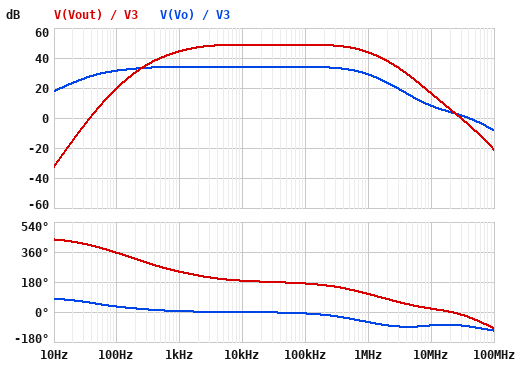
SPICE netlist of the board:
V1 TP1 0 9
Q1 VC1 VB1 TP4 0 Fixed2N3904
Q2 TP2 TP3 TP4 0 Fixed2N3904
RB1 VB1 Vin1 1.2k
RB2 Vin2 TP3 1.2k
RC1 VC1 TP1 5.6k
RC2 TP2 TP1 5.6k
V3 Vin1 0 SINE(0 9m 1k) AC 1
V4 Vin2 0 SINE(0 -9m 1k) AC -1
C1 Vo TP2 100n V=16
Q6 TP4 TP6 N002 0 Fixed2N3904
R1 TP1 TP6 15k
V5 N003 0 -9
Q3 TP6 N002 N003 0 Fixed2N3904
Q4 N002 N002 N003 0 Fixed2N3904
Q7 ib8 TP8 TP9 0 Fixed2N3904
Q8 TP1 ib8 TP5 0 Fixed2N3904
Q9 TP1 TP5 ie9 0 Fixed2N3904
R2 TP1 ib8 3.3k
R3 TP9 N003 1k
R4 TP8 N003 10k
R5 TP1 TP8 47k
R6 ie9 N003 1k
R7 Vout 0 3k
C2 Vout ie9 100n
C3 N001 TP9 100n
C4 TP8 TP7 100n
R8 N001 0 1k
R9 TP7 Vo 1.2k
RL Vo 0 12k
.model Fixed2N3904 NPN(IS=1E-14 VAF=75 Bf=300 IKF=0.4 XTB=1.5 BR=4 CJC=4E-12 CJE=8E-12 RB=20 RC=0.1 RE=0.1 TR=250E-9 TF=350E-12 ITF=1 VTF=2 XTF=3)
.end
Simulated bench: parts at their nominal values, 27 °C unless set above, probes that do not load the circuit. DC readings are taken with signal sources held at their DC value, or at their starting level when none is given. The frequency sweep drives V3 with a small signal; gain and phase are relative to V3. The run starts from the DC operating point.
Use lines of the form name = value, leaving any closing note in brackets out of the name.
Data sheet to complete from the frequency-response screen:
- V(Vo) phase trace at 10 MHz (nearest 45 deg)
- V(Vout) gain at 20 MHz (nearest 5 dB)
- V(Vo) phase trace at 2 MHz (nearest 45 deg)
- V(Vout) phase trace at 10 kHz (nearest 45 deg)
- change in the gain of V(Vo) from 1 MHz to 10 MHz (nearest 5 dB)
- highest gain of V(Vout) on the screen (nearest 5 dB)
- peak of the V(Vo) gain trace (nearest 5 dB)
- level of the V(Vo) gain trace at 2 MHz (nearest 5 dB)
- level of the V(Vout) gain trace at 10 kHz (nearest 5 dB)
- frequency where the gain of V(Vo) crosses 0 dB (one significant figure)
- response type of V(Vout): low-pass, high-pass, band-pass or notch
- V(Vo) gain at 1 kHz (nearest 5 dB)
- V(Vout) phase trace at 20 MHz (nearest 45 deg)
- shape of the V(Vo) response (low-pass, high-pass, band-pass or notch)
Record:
V(Vo) phase trace at 10 MHz = -90 deg
V(Vout) gain at 20 MHz = 5 dB
V(Vo) phase trace at 2 MHz = -90 deg
V(Vout) phase trace at 10 kHz = 180 deg
change in the gain of V(Vo) from 1 MHz to 10 MHz = -20 dB
highest gain of V(Vout) on the screen = 50 dB
peak of the V(Vo) gain trace = 35 dB
level of the V(Vo) gain trace at 2 MHz = 25 dB
level of the V(Vout) gain trace at 10 kHz = 50 dB
frequency where the gain of V(Vo) crosses 0 dB = 40 MHz
response type of V(Vout): low-pass, high-pass, band-pass or notch = band-pass
V(Vo) gain at 1 kHz = 35 dB
V(Vout) phase trace at 20 MHz = 0 deg
shape of the V(Vo) response = band-pass
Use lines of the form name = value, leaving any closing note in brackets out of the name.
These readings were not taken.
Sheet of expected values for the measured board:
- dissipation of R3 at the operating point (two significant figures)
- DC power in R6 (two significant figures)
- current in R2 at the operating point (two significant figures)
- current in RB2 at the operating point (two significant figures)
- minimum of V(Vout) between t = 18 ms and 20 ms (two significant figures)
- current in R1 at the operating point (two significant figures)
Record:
dissipation of R3 at the operating point = 5.9 mW
DC power in R6 = 77 mW
current in R2 at the operating point = 2.4 mA
current in RB2 at the operating point = 1.7 µA
minimum of V(Vout) between t = 18 ms and 20 ms = -1.5 V
current in R1 at the operating point = 1.1 mA
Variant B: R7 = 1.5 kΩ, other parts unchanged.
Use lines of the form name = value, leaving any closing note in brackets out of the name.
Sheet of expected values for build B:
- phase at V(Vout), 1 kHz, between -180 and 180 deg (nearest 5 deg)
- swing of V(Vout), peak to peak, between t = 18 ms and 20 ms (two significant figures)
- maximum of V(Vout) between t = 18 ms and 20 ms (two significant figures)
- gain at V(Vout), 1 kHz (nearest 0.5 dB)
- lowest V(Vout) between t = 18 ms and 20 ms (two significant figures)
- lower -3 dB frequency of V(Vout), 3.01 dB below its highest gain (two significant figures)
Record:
phase at V(Vout), 1 kHz, between -180 and 180 deg = -100 deg
swing of V(Vout), peak to peak, between t = 18 ms and 20 ms = 2.3 V
maximum of V(Vout) between t = 18 ms and 20 ms = 1.2 V
gain at V(Vout), 1 kHz = 42.5 dB
lowest V(Vout) between t = 18 ms and 20 ms = -1.2 V
lower -3 dB frequency of V(Vout), 3.01 dB below its highest gain = 1.8 kHz
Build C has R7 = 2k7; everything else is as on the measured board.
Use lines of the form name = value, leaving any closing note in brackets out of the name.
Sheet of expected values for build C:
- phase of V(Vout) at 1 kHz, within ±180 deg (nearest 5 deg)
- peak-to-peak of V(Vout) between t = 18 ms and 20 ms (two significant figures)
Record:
phase of V(Vout) at 1 kHz, within ±180 deg = -115 deg
peak-to-peak of V(Vout) between t = 18 ms and 20 ms = 2.9 V
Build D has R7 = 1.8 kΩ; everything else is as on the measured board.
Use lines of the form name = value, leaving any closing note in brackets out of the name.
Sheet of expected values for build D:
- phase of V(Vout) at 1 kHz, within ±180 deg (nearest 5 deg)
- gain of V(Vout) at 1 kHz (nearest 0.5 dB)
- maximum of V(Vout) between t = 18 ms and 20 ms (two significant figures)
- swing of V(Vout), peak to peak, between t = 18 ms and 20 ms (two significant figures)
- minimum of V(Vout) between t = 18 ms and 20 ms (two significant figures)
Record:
phase of V(Vout) at 1 kHz, within ±180 deg = -105 deg
gain of V(Vout) at 1 kHz = 43.0 dB
maximum of V(Vout) between t = 18 ms and 20 ms = 1.3 V
swing of V(Vout), peak to peak, between t = 18 ms and 20 ms = 2.5 V
minimum of V(Vout) between t = 18 ms and 20 ms = -1.3 V
